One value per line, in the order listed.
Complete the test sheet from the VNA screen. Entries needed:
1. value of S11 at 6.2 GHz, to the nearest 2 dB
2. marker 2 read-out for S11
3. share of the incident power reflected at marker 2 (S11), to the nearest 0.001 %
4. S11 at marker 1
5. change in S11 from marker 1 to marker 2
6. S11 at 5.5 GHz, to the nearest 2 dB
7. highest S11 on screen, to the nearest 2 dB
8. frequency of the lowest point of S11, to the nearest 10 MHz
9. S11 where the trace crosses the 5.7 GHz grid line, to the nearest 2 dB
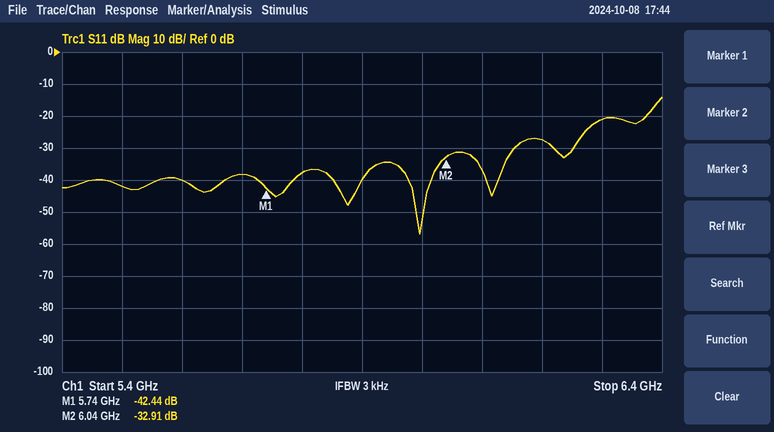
-28 dB
-32.91 dB
0.051 %
-42.44 dB
9.53 dB
-42 dB
-14 dB
6.00 GHz
-38 dB
